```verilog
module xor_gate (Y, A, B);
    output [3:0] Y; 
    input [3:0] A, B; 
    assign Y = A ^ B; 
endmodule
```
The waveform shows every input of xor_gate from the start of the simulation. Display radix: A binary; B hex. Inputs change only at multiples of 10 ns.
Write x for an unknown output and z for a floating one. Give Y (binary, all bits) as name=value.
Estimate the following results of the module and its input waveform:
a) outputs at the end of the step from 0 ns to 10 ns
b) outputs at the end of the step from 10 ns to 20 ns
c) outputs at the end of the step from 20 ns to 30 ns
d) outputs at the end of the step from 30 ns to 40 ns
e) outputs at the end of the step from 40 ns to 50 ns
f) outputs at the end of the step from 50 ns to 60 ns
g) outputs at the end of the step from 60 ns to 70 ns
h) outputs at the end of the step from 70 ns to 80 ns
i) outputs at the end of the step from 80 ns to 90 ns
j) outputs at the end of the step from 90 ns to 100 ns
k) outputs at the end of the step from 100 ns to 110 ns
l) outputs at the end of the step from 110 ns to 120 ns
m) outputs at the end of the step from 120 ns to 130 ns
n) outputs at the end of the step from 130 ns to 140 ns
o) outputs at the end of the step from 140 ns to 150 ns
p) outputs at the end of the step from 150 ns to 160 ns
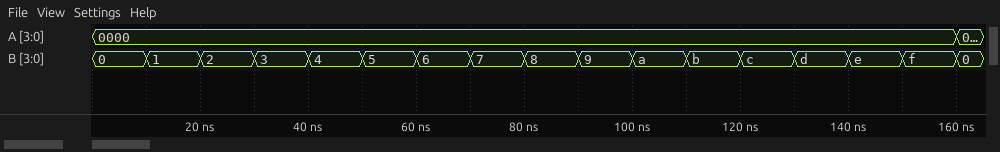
Y=0000
Y=0001
Y=0010
Y=0011
Y=0100
Y=0101
Y=0110
Y=0111
Y=1000
Y=1001
Y=1010
Y=1011
Y=1100
Y=1101
Y=1110
Y=1111
